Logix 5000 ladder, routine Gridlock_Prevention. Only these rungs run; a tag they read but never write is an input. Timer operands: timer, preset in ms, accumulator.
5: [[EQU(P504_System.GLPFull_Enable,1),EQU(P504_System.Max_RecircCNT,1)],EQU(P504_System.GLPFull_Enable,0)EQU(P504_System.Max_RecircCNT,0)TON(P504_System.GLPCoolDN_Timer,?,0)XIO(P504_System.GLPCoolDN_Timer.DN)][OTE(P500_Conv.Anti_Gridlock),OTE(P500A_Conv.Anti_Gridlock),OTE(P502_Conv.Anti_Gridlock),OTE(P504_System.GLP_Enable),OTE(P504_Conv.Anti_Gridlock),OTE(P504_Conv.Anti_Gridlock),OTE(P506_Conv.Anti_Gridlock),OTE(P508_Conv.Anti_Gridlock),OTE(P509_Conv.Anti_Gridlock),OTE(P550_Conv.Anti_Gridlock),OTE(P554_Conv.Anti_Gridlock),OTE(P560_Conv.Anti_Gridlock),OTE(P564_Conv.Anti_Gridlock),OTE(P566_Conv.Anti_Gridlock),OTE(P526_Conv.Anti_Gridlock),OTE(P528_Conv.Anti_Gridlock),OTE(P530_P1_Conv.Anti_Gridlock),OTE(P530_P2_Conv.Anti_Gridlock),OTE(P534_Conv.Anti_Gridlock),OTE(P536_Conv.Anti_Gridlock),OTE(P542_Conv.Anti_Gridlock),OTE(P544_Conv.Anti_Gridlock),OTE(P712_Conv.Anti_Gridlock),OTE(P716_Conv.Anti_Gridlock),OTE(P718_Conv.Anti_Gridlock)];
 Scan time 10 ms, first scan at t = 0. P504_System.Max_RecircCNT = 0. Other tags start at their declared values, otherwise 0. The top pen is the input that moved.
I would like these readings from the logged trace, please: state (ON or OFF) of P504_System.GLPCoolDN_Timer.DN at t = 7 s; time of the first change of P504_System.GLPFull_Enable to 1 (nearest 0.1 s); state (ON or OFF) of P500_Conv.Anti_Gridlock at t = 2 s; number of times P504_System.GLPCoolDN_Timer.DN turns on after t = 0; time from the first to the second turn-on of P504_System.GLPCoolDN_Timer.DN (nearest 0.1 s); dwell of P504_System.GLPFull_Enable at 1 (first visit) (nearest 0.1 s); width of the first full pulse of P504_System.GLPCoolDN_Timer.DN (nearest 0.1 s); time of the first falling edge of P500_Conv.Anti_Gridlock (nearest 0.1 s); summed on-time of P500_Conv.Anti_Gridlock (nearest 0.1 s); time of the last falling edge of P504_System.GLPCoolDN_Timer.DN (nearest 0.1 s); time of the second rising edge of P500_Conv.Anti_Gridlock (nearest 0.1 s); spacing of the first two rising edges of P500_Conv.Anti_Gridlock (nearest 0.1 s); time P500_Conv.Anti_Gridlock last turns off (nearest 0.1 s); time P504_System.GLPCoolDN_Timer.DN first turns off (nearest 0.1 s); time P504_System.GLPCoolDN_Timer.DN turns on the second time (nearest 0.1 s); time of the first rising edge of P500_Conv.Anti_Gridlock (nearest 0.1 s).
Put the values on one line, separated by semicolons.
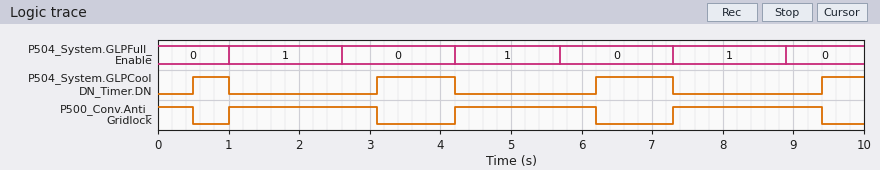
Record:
ON; 1.0 s; ON; 4; 2.6 s; 1.6 s; 0.5 s; 0.5 s; 6.7 s; 7.3 s; 4.2 s; 3.2 s; 9.4 s; 1.0 s; 3.1 s; 1.0 s
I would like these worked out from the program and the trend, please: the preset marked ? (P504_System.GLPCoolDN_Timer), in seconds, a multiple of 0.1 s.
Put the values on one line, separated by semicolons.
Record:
0.5 s
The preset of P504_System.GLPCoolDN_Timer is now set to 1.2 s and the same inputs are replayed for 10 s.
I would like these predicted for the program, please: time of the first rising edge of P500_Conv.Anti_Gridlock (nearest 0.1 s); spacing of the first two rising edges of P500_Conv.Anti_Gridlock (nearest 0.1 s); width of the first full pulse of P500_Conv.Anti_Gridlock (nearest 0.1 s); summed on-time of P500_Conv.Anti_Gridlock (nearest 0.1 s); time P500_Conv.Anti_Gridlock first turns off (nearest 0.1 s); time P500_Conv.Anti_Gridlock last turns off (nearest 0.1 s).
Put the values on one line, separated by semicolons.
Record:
4.2 s; 3.1 s; 2.7 s; 9.2 s; 3.8 s; 6.9 s
